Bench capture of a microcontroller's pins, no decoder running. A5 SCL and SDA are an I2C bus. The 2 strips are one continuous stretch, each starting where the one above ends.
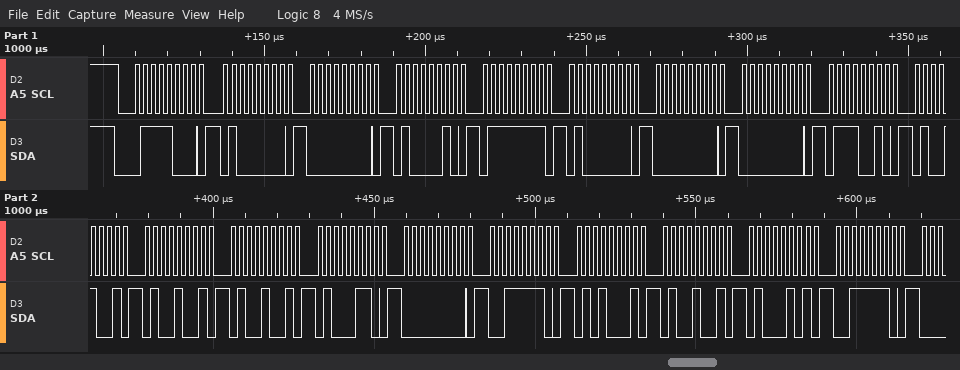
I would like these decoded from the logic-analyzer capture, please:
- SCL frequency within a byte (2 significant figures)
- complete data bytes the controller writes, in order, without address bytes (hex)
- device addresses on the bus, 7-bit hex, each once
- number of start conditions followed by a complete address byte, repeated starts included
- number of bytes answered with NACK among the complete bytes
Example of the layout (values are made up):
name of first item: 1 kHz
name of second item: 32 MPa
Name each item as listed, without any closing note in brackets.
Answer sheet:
SCL frequency within a byte: 400 kHz
complete data bytes the controller writes, in order, without address bytes: 40 00 42 7F 40 00 00 72 49 49 49 46 00 3E 51 49 45 3E
device addresses on the bus, 7-bit hex, each once: 0x3C
number of start conditions followed by a complete address byte, repeated starts included: 1
number of bytes answered with NACK among the complete bytes: 0
